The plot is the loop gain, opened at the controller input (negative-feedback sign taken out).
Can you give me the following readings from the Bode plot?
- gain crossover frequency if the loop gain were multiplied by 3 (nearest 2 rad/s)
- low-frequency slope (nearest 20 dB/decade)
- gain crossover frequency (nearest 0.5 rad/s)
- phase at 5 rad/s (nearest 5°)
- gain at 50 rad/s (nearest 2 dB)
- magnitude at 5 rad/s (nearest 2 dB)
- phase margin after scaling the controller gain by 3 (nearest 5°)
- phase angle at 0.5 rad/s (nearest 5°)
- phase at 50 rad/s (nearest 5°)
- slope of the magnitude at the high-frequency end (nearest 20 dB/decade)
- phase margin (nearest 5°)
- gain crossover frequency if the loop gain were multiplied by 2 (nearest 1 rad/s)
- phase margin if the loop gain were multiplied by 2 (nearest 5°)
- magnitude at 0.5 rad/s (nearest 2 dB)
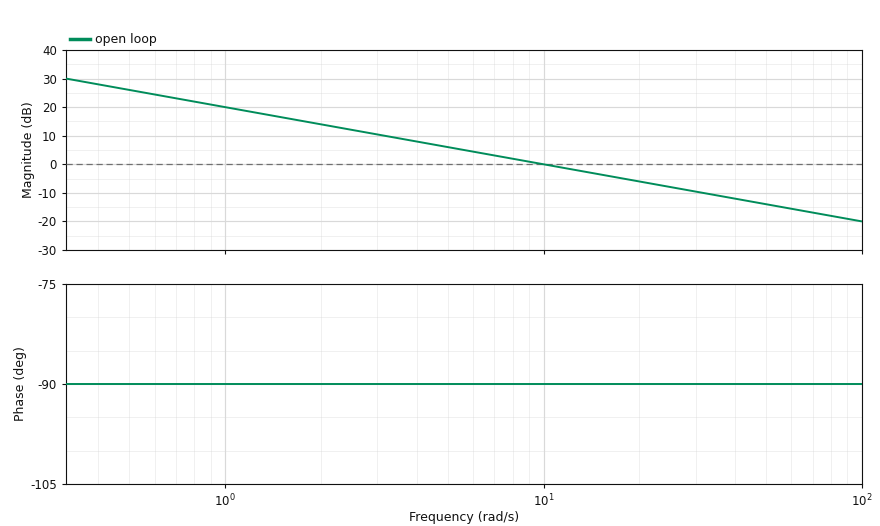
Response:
30 rad/s
-20 dB/decade
10.0 rad/s
-90°
-14 dB
6 dB
90°
-90°
-90°
-20 dB/decade
90°
20 rad/s
90°
26 dB
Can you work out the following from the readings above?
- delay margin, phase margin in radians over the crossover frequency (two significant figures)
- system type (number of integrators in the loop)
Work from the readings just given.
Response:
0.16 s
1
